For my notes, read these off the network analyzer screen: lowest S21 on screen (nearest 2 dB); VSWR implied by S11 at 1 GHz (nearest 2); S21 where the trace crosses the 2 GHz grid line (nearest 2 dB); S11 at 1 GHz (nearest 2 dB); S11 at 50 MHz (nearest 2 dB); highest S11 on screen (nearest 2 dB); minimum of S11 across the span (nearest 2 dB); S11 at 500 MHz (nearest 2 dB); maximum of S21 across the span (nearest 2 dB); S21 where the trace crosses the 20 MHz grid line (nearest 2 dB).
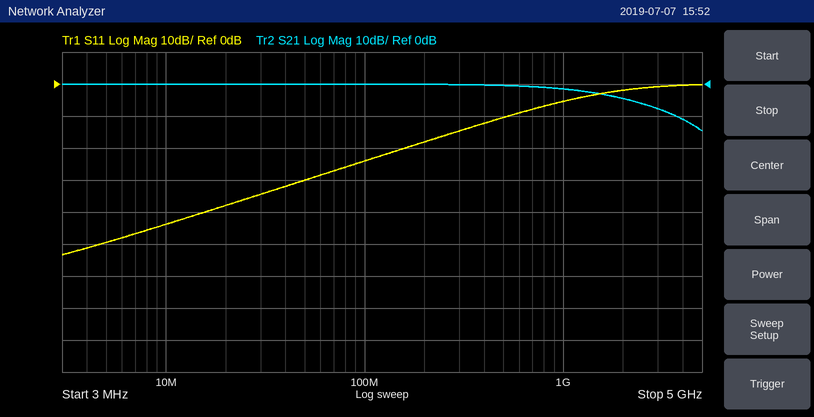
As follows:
-14 dB
4
-4 dB
-6 dB
-30 dB
0 dB
-54 dB
-10 dB
0 dB
0 dB
